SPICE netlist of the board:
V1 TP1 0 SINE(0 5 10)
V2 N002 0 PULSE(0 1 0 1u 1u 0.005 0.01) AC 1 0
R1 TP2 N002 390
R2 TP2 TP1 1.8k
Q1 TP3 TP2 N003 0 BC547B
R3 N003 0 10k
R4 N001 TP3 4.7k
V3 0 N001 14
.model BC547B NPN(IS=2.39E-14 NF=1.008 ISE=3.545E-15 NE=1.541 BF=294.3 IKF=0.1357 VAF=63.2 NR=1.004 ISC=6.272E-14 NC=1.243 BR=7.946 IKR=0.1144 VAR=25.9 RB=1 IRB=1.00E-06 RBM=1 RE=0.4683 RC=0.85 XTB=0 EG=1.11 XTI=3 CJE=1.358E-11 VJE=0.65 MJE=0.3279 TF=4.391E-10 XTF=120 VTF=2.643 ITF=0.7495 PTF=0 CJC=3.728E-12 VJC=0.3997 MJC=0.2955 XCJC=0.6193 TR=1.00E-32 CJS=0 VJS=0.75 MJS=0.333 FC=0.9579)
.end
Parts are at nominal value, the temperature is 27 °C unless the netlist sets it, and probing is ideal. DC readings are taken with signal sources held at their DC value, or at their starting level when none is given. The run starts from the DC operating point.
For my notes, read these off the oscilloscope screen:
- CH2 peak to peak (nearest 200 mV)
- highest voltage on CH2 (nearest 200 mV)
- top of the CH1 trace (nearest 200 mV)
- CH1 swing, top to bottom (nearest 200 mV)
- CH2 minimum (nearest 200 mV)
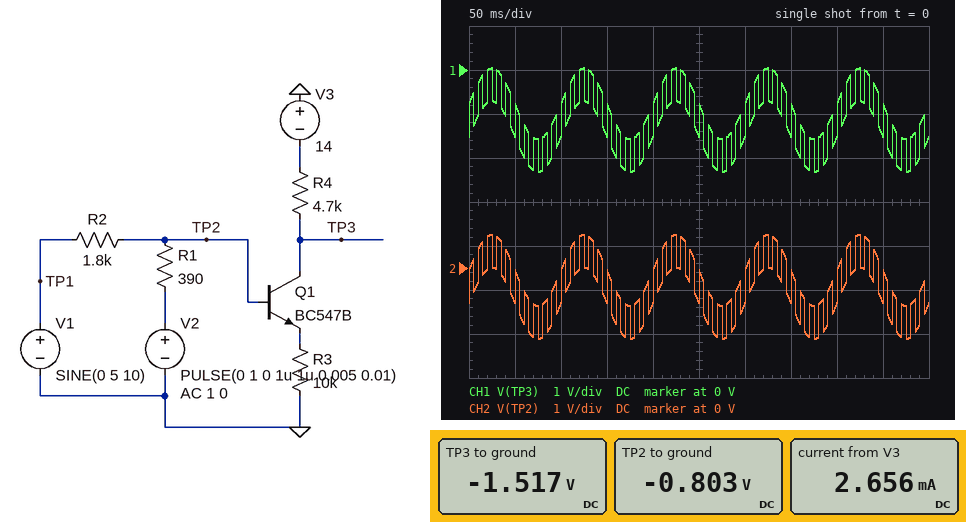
2.4 V
800 mV
0 V
2.4 V
-1.6 V
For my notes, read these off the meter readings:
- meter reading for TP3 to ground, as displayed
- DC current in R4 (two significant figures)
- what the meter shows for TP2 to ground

-1.517 V
2.7 mA
-0.803 V
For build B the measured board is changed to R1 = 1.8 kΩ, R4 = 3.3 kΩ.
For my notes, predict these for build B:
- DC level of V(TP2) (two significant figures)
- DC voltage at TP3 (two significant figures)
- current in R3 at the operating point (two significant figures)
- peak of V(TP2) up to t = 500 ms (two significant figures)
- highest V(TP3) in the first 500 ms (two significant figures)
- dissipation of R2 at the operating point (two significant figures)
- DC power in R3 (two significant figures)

-2.6 V
-3.3 V
330 µA
-410 mV
-1.1 V
3.8 mW
1.1 mW
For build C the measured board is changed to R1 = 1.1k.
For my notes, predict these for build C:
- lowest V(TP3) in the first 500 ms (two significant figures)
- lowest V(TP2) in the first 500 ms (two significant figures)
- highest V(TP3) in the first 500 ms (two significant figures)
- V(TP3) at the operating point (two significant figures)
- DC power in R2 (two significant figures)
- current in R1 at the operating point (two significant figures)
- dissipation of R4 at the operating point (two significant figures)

-3.8 V
-3.1 V
-190 mV
-2.3 V
1.3 mW
1.4 mA
29 mW
